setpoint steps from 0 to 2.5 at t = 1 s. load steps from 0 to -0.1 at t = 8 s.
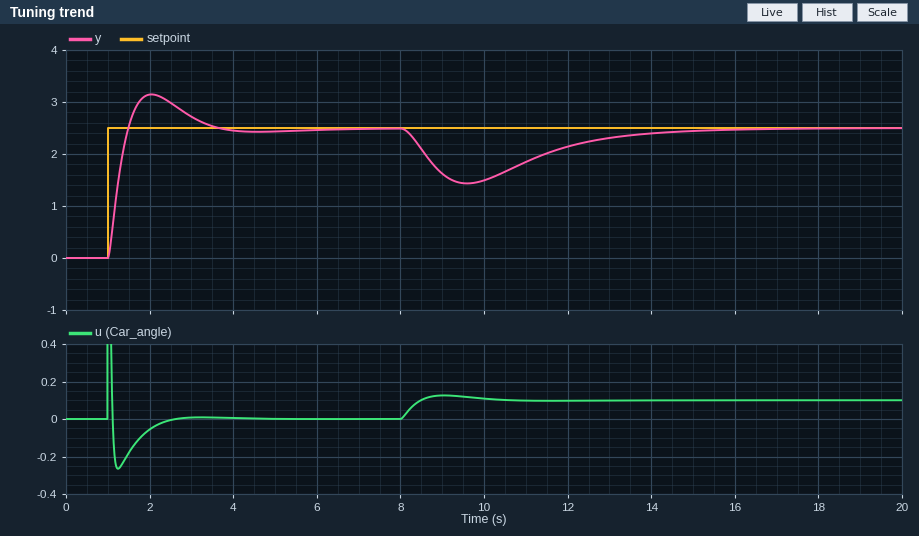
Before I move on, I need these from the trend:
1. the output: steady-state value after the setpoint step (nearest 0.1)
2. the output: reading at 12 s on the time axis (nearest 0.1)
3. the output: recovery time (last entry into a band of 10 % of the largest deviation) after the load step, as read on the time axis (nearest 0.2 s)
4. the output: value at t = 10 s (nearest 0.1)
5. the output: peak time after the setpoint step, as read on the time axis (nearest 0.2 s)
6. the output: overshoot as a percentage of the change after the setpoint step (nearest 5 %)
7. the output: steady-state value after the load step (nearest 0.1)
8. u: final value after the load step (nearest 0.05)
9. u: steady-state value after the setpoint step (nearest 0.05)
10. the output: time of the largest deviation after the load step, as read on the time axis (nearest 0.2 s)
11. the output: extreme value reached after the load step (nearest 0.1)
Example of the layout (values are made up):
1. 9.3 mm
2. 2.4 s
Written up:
1. 2.5
2. 2.1
3. 14.0 s
4. 1.5
5. 2.0 s
6. 25 %
7. 2.5
8. 0.10
9. 0.00
10. 9.6 s
11. 1.4
